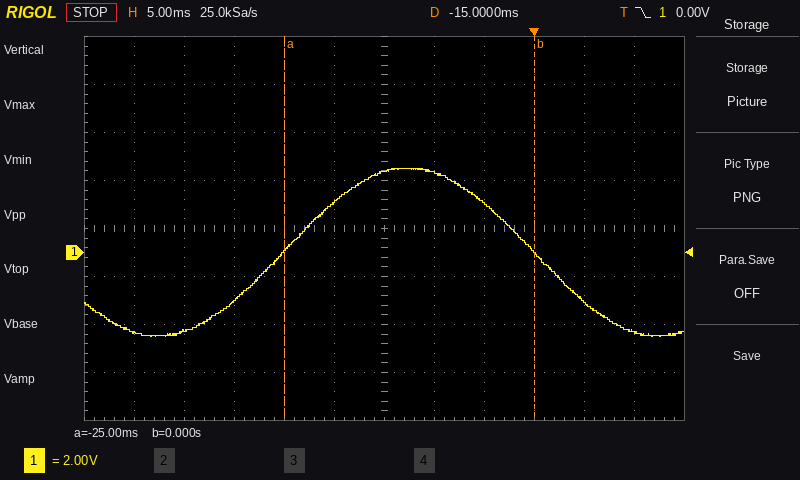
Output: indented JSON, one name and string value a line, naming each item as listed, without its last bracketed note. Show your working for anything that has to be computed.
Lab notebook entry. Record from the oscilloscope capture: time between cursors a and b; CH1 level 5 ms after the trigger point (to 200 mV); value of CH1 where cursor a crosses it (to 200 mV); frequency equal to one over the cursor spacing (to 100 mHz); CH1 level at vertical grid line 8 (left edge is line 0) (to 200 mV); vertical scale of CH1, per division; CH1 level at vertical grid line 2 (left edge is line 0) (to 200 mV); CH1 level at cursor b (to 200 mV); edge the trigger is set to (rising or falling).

{
  "time between cursors a and b": "0 s − (-25 ms) = 25.0 ms",
  "CH1 level 5 ms after the trigger point": "-2.0 V",
  "value of CH1 where cursor a crosses it": "0.0 V",
  "frequency equal to one over the cursor spacing": "1 / 25.0 ms ≈ 40.0 Hz",
  "CH1 level at vertical grid line 8 (left edge is line 0)": "2.0 V",
  "vertical scale of CH1, per division": "2 V",
  "CH1 level at vertical grid line 2 (left edge is line 0)": "-3.2 V",
  "CH1 level at cursor b": "0.0 V",
  "edge the trigger is set to": "falling"
}
